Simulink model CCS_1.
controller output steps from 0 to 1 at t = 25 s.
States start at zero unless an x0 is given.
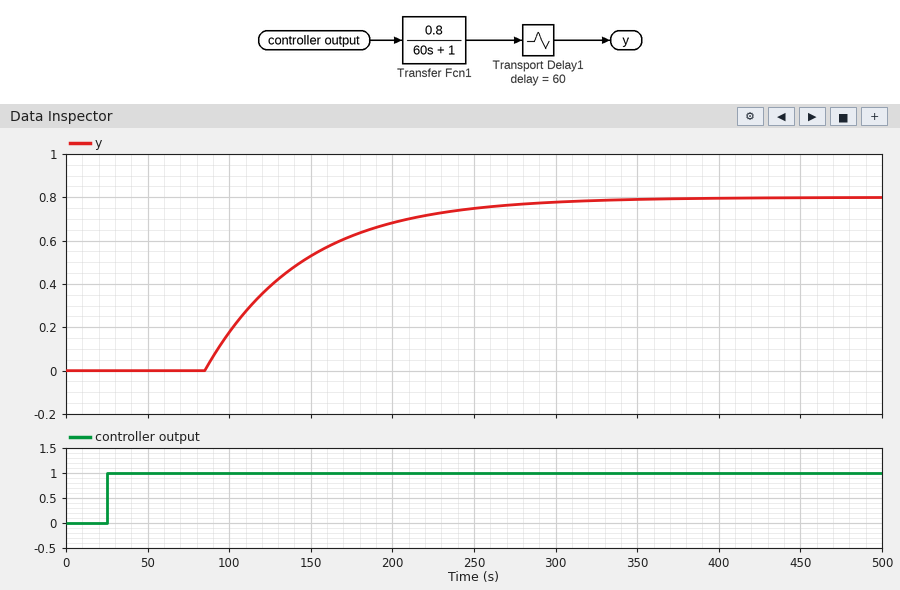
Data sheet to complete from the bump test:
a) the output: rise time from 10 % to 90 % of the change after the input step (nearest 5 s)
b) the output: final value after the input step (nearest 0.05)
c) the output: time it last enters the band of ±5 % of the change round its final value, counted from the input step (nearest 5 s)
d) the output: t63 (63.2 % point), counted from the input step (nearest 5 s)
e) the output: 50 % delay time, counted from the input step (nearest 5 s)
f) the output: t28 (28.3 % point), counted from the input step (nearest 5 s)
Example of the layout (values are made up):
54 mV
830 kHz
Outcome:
130 s
0.80
240 s
120 s
100 s
80 s
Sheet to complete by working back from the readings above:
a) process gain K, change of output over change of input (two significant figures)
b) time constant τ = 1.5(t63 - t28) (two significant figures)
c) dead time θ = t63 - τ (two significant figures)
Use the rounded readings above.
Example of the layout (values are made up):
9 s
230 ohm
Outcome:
0.80
60 s
60 s
